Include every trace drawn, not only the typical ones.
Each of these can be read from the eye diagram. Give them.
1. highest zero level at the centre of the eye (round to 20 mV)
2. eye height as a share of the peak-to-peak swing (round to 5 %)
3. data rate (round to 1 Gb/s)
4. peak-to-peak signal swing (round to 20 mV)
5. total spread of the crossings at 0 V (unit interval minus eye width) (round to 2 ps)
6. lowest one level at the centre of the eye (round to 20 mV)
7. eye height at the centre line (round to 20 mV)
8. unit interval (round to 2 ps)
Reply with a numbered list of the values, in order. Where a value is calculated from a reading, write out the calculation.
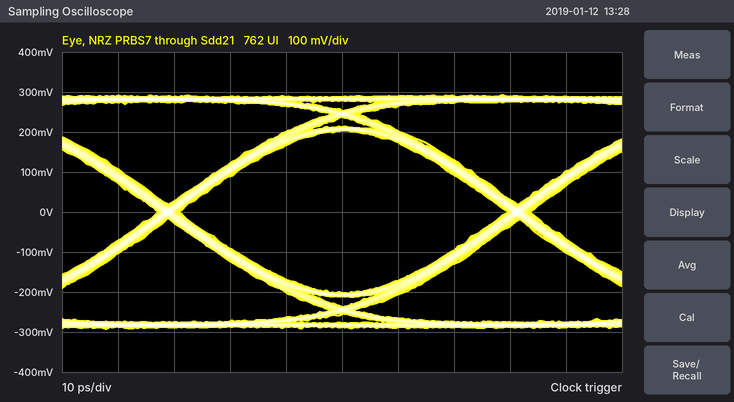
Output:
1. -200 mV
2. 400 mV / 580 mV ≈ 69.0 %, so 70 % to the nearest 5 %
3. 16 Gb/s
4. 580 mV
5. 4 ps
6. 200 mV
7. 400 mV
8. 62 ps
